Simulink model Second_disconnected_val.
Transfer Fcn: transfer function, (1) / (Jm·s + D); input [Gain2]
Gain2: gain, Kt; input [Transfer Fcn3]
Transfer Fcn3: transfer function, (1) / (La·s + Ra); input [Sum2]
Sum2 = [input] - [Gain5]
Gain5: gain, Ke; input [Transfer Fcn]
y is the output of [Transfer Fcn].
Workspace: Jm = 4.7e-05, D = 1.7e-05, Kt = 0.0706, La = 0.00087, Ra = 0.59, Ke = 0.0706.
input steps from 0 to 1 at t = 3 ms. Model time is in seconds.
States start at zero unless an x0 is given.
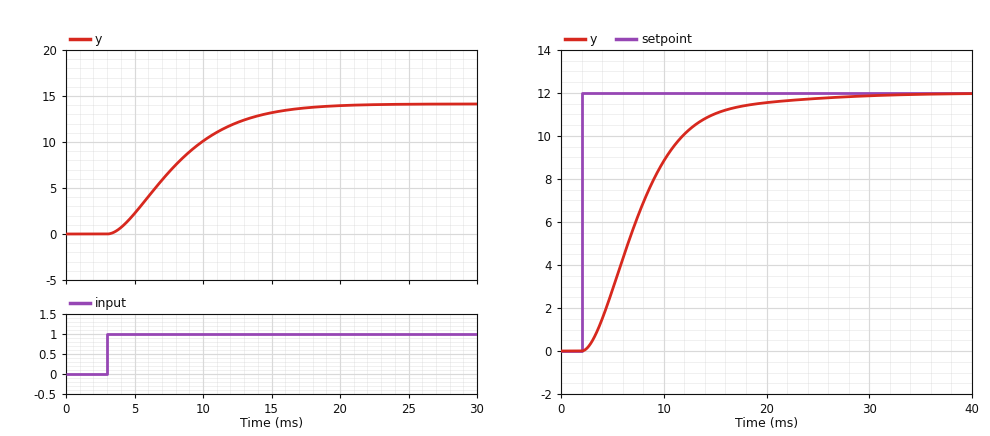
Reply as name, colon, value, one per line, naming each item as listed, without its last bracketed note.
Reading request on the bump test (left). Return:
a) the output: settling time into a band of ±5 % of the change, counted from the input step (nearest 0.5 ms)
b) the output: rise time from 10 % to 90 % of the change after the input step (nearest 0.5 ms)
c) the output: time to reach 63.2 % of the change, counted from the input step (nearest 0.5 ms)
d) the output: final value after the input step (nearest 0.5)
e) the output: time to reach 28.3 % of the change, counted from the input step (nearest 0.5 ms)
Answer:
the output: settling time into a band of ±5 % of the change, counted from the input step: 13.0 ms
the output: rise time from 10 % to 90 % of the change after the input step: 9.0 ms
the output: time to reach 63.2 % of the change, counted from the input step: 6.0 ms
the output: final value after the input step: 14.0
the output: time to reach 28.3 % of the change, counted from the input step: 3.0 ms
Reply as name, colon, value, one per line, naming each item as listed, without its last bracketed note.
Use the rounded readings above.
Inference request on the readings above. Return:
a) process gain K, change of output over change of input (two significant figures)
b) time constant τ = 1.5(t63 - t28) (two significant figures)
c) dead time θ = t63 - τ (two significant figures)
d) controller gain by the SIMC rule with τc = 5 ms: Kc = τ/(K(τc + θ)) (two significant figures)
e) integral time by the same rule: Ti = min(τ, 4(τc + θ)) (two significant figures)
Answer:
process gain K, change of output over change of input: 14
time constant τ = 1.5(t63 - t28): 4.5 ms
dead time θ = t63 - τ: 1.5 ms
controller gain by the SIMC rule with τc = 5 ms: Kc = τ/(K(τc + θ)): 0.049
integral time by the same rule: Ti = min(τ, 4(τc + θ)): 4.5 ms
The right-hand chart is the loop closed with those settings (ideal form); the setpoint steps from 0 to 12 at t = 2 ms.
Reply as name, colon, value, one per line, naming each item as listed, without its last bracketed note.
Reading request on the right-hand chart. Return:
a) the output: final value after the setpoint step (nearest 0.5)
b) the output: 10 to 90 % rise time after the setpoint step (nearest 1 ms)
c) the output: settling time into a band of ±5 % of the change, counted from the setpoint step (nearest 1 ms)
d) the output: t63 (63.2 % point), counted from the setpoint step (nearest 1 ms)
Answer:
the output: final value after the setpoint step: 12.0
the output: 10 to 90 % rise time after the setpoint step: 10 ms
the output: settling time into a band of ±5 % of the change, counted from the setpoint step: 16 ms
the output: t63 (63.2 % point), counted from the setpoint step: 7 ms
